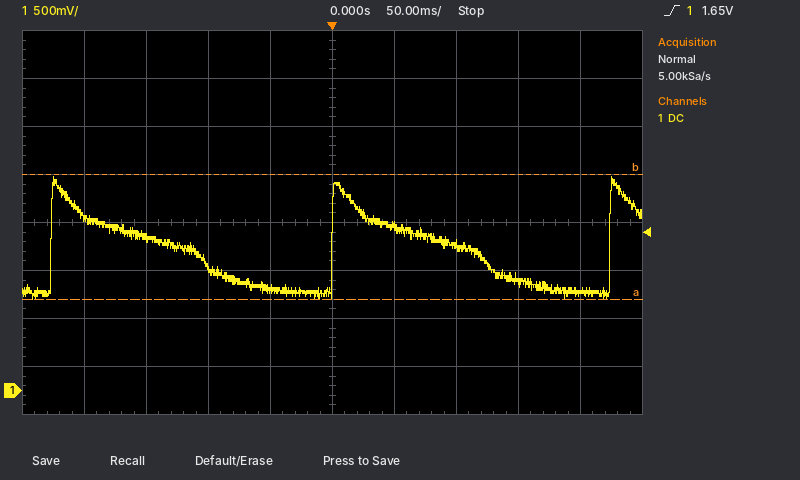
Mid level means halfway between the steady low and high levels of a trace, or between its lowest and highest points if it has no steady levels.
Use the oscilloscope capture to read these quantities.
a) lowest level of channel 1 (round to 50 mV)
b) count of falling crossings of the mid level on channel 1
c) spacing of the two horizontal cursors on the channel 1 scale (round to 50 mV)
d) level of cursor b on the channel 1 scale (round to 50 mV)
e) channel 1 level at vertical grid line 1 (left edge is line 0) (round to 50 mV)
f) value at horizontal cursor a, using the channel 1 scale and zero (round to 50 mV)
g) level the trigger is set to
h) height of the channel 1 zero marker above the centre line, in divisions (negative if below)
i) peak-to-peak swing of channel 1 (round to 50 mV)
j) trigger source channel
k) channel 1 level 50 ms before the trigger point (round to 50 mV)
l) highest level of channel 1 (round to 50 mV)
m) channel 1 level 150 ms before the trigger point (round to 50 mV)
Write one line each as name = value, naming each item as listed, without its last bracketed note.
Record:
lowest level of channel 1 = 950 mV
count of falling crossings of the mid level on channel 1 = 2
spacing of the two horizontal cursors on the channel 1 scale = 1.30 V
level of cursor b on the channel 1 scale = 2.25 V
channel 1 level at vertical grid line 1 (left edge is line 0) = 1.80 V
value at horizontal cursor a, using the channel 1 scale and zero = 950 mV
level the trigger is set to = 1.65 V
height of the channel 1 zero marker above the centre line, in divisions = -3.5 div
peak-to-peak swing of channel 1 = 1.30 V
trigger source channel = channel 1
channel 1 level 50 ms before the trigger point = 1.05 V
highest level of channel 1 = 2.25 V
channel 1 level 150 ms before the trigger point = 1.60 V
